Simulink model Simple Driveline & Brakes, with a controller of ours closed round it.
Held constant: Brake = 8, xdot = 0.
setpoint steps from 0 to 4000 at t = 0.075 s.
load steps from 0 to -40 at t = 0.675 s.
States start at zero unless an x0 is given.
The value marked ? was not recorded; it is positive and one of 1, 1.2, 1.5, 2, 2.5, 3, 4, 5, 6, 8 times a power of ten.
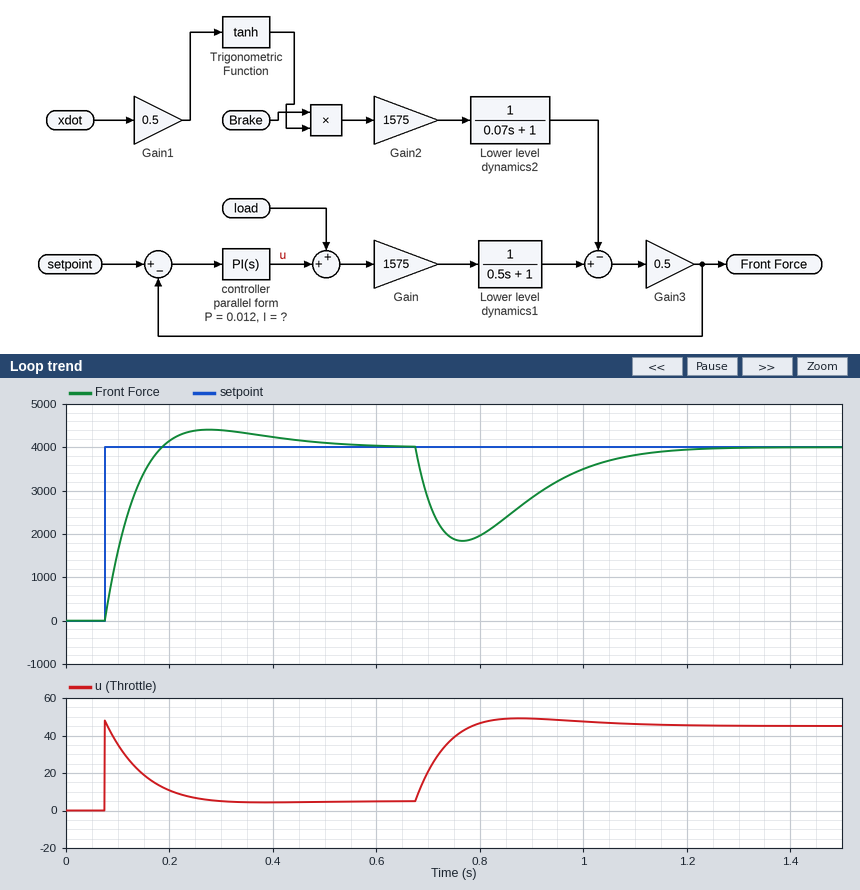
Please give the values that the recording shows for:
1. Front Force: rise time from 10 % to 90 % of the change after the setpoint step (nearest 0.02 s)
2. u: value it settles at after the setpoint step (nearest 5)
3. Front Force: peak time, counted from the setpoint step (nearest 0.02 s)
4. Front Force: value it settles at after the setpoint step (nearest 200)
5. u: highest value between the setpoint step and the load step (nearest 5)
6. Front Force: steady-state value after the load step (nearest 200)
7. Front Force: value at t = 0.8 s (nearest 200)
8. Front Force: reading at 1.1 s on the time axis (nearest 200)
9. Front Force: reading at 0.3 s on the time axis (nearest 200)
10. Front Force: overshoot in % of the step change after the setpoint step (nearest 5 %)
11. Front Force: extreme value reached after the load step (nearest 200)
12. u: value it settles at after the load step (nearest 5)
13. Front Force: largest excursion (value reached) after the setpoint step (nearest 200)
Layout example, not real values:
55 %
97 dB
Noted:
0.08 s
5
0.20 s
4000
50
4000
2000
3800
4400
10 %
1800
45
4400
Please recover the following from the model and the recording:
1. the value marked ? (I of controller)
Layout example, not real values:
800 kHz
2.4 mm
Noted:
0.08
